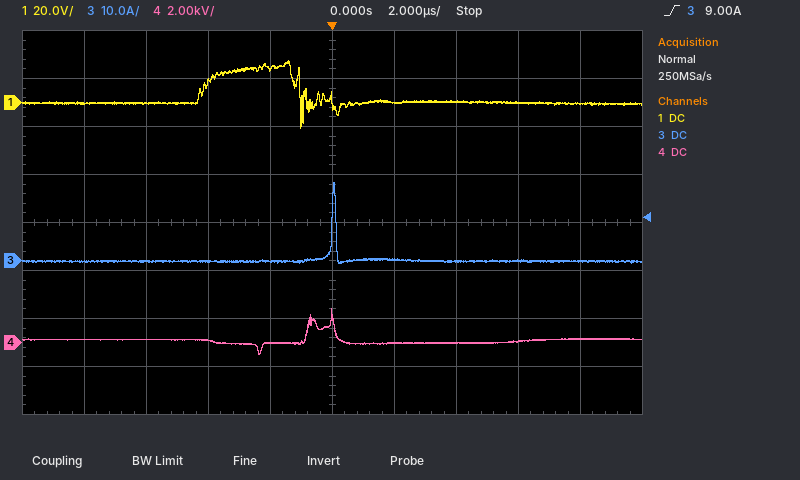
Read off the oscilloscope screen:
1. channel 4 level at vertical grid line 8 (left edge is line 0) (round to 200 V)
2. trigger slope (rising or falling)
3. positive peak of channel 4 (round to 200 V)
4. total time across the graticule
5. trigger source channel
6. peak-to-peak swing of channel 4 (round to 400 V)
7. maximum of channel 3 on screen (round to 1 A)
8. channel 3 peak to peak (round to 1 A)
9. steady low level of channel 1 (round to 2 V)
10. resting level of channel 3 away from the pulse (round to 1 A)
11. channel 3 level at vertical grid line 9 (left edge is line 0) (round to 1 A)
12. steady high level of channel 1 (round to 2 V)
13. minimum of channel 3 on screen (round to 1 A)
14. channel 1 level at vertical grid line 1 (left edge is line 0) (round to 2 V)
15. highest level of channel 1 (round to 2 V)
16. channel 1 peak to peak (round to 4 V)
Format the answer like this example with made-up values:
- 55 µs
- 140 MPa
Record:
- 0.0 kV
- rising
- 1.4 kV
- 20 µs
- channel 3
- 2.0 kV
- 16 A
- 17 A
- 0 V
- 0 A
- 0 A
- 14 V
- -1 A
- 0 V
- 18 V
- 28 V
